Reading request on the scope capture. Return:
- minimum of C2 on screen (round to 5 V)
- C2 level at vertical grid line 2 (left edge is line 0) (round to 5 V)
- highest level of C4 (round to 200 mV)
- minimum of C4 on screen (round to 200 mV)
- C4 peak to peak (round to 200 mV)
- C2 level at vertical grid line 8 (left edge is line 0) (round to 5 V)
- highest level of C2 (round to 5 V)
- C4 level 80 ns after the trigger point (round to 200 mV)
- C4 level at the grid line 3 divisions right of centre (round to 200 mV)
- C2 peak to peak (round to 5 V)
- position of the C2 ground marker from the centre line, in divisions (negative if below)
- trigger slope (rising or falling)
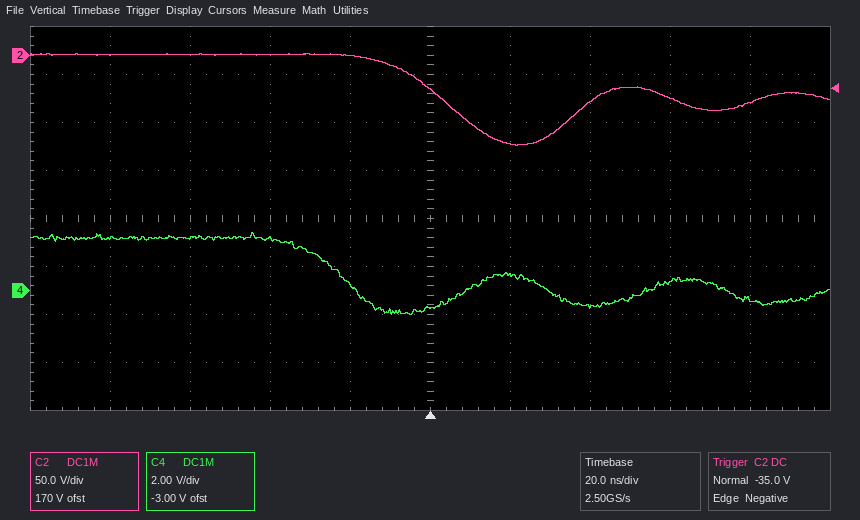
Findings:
-95 V
0 V
2.4 V
-1.0 V
3.4 V
-45 V
0 V
-400 mV
400 mV
95 V
+3.4 div
falling
